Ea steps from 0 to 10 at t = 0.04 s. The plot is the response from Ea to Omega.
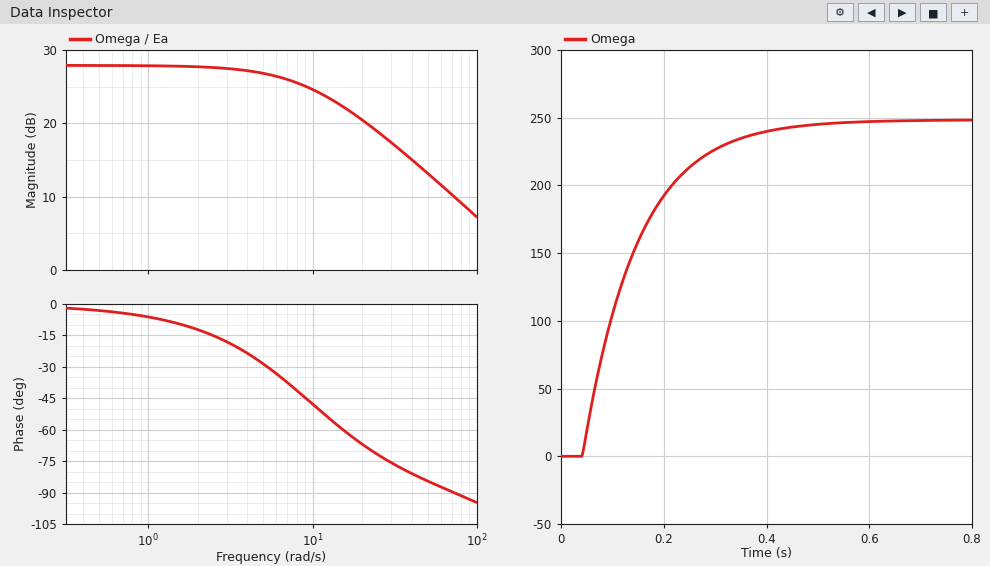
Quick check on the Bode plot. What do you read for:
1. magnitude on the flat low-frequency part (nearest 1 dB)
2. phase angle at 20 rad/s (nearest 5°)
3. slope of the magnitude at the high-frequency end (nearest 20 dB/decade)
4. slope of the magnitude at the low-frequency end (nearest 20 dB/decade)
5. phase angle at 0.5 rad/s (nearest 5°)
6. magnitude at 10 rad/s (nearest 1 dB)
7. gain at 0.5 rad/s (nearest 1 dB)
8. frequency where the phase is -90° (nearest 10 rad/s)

28 dB
-65°
-20 dB/decade
0 dB/decade
-5°
25 dB
28 dB
70 rad/s
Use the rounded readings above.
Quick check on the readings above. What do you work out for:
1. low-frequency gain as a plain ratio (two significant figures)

25
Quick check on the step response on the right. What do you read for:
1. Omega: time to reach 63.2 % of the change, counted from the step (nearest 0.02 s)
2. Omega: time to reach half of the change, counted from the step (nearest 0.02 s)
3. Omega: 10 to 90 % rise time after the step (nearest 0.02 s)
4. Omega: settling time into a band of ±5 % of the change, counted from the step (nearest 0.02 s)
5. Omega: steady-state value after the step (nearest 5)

0.10 s
0.08 s
0.24 s
0.32 s
250
